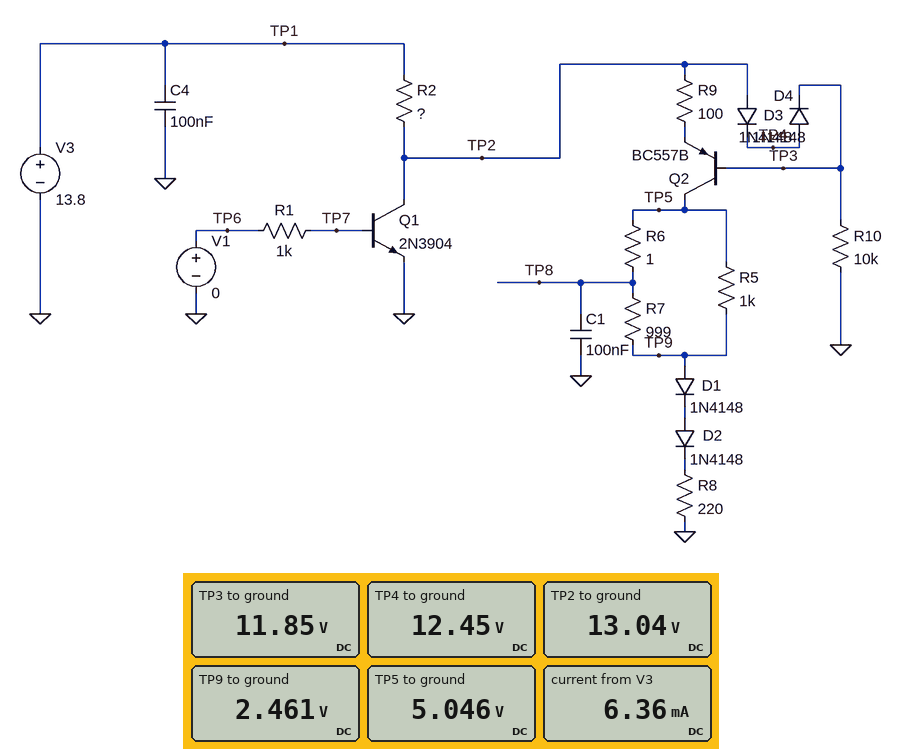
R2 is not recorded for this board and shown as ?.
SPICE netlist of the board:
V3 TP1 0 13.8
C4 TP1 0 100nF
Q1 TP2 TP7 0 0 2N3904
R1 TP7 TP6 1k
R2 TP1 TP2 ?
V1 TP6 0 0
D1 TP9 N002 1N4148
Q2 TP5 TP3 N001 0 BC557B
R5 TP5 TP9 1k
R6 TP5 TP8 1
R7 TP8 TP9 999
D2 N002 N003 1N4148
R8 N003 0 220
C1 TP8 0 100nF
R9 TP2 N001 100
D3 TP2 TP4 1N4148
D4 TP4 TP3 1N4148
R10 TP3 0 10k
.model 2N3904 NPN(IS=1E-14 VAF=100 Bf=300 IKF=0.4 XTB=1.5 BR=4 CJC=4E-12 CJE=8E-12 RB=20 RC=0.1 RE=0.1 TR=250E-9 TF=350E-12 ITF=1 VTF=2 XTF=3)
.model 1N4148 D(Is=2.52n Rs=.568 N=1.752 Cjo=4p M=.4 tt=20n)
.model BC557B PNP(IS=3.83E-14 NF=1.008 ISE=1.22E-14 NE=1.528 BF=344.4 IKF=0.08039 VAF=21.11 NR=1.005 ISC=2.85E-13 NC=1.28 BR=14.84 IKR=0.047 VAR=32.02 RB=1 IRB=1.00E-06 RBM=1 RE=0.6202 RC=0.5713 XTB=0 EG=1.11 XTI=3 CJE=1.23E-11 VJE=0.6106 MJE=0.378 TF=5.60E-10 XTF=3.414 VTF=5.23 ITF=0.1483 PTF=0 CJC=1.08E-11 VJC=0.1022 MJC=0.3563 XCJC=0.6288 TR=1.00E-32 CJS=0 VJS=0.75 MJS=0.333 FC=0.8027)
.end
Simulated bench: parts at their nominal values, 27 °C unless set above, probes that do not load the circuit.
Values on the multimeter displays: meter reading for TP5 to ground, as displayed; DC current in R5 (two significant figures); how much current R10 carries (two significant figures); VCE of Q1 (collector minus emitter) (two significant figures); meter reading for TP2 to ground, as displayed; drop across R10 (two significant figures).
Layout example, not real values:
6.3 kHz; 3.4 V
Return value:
5.046 V; 2.6 mA; 1.2 mA; 13 V; 13.04 V; 12 V
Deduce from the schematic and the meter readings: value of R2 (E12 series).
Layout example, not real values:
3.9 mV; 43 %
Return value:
120 Ω
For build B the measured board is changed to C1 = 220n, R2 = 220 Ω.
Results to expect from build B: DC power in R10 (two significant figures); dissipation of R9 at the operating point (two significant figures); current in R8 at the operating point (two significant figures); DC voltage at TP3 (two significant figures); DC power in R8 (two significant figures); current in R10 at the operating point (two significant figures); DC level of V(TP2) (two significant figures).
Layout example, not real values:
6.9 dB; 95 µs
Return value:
13 mW; 2.6 mW; 5.1 mA; 11 V; 5.8 mW; 1.1 mA; 12 V
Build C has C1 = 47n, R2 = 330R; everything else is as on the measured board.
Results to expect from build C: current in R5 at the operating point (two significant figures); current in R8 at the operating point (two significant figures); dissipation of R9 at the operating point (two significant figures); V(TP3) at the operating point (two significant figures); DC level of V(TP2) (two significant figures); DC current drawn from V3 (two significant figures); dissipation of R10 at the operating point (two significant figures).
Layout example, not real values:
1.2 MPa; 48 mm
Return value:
2.5 mA; 5.1 mA; 2.6 mW; 11 V; 12 V; 6.1 mA; 11 mW
